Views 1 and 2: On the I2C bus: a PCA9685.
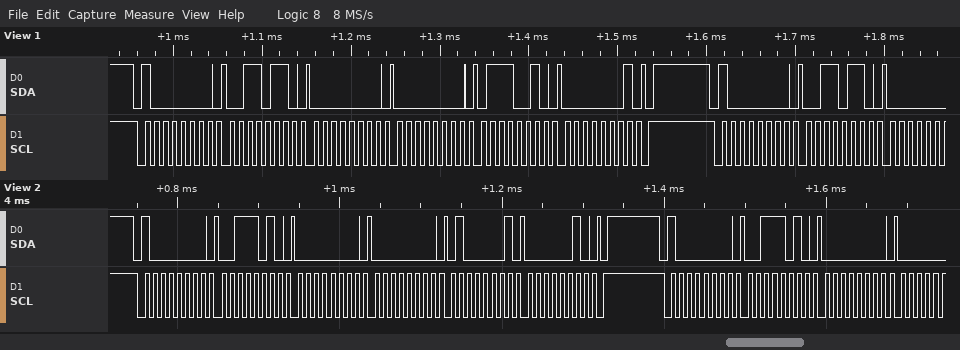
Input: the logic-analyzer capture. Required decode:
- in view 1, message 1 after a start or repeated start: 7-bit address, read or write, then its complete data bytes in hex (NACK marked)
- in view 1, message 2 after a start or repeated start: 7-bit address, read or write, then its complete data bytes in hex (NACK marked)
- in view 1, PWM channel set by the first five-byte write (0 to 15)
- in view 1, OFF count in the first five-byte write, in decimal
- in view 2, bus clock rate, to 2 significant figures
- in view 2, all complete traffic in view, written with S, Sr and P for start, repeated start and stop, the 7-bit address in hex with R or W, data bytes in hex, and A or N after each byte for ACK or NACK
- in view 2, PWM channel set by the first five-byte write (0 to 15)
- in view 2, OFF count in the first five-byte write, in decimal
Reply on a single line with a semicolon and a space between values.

0x40 write: 36 00 00 72 01; 0x40 write: 36; 12; 370; 100 kHz; S 40W A 3A A 00 A 00 A 41 A 02 A P S 40W A 3A A 00 A; 13; 577
